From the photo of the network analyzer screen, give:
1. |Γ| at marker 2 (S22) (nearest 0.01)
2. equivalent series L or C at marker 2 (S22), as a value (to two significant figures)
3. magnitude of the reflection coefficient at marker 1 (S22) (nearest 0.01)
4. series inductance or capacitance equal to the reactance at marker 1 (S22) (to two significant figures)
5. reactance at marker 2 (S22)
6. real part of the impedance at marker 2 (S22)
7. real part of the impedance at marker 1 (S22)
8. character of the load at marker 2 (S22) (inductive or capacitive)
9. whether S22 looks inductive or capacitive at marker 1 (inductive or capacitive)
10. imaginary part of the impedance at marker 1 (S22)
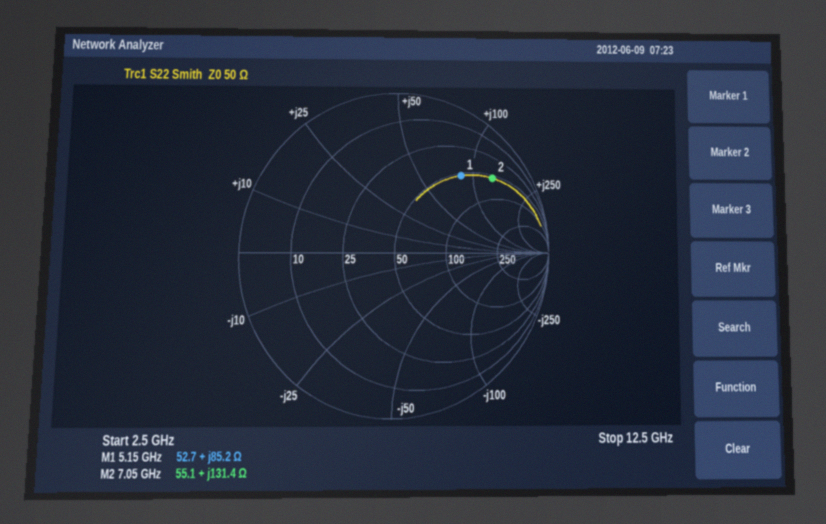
0.78
3.0 nH
0.64
2.6 nH
+131.4 Ω
55.1 Ω
52.7 Ω
inductive
inductive
+85.2 Ω
